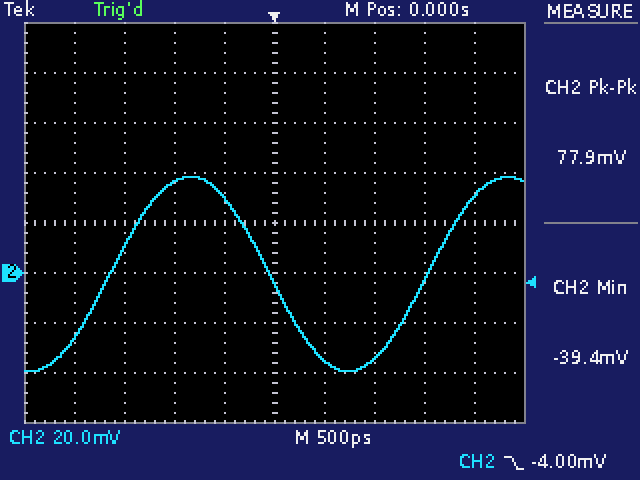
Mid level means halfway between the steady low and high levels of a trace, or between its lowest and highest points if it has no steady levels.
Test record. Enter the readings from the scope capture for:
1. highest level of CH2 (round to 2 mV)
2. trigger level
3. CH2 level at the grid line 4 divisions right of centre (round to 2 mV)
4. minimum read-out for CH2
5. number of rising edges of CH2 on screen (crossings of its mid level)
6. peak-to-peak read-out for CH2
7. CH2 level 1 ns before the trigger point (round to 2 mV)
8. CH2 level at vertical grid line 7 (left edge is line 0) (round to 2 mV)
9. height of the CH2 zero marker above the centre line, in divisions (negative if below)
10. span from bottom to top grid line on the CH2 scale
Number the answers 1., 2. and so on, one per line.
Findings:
1. 38 mV
2. -4.00 mV
3. 30 mV
4. -39.4 mV
5. 2
6. 77.9 mV
7. 36 mV
8. -34 mV
9. -1.0 div
10. 160 mV
